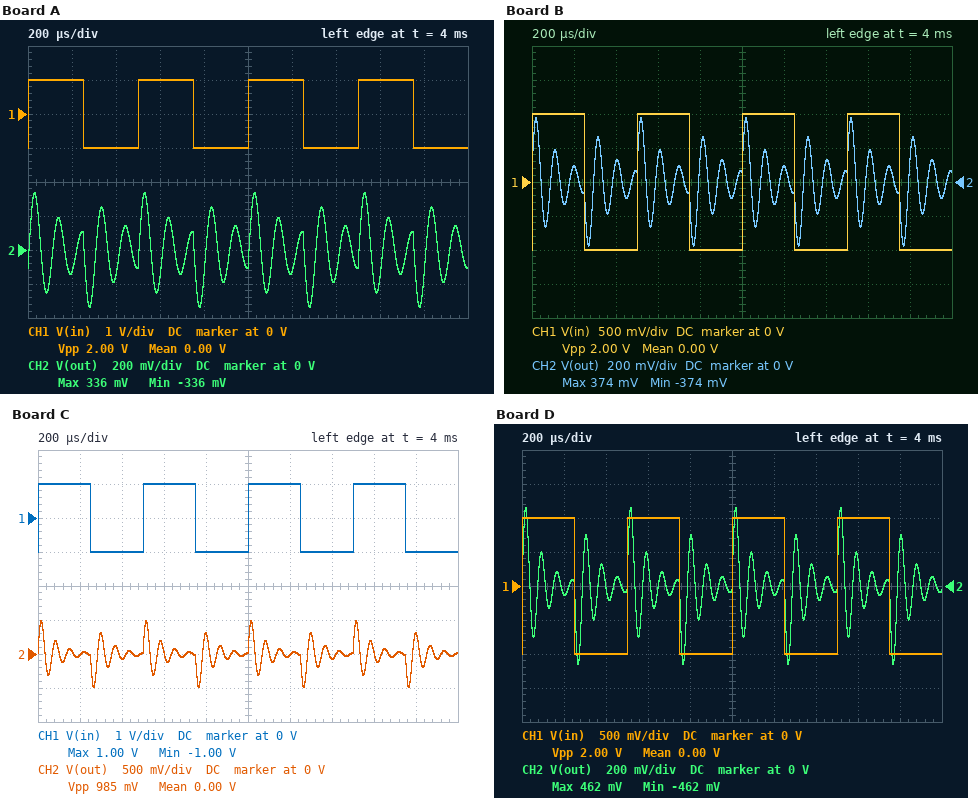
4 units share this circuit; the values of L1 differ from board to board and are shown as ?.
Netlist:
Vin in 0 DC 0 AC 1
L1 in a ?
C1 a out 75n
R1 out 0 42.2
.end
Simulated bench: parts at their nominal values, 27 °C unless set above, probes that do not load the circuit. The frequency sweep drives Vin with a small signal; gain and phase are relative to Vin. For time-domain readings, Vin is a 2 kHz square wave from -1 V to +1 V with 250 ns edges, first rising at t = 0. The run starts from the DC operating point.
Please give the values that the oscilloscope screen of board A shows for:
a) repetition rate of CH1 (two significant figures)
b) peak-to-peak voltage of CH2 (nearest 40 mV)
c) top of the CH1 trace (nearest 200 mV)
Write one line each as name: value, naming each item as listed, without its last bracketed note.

repetition rate of CH1: 2.0 kHz
peak-to-peak voltage of CH2: 680 mV
top of the CH1 trace: 1.0 V
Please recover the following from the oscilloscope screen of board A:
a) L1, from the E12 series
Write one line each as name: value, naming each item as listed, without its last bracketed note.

L1, from the E12 series: 3.9 mH
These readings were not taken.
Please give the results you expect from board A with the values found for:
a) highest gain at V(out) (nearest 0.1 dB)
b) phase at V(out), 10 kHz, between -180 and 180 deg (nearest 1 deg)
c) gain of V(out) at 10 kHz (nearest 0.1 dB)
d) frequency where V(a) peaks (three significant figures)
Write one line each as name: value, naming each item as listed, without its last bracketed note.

highest gain at V(out): 0 dB
phase at V(out), 10 kHz, between -180 and 180 deg: -38 deg
gain of V(out) at 10 kHz: -2.1 dB
frequency where V(a) peaks: 9.23 kHz
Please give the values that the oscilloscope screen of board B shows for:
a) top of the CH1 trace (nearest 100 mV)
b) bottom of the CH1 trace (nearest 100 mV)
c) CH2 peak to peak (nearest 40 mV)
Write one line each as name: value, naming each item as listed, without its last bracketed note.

top of the CH1 trace: 1.0 V
bottom of the CH1 trace: -1.0 V
CH2 peak to peak: 760 mV
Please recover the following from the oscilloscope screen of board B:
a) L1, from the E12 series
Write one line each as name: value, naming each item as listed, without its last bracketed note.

L1, from the E12 series: 2.7 mH
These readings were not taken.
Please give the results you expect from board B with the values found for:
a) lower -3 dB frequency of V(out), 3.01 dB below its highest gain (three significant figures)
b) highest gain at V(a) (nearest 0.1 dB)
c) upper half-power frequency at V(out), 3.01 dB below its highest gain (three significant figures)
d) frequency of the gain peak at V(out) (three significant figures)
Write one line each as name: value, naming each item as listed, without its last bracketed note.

lower -3 dB frequency of V(out), 3.01 dB below its highest gain: 10.0 kHz
highest gain at V(a): 13.3 dB
upper half-power frequency at V(out), 3.01 dB below its highest gain: 12.5 kHz
frequency of the gain peak at V(out): 11.2 kHz
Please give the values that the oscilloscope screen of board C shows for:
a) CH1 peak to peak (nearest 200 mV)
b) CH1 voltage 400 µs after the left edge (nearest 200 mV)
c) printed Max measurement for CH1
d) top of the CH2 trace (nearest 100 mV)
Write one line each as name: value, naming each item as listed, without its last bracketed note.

CH1 peak to peak: 2.0 V
CH1 voltage 400 µs after the left edge: -1.0 V
printed Max measurement for CH1: 1.00 V
top of the CH2 trace: 500 mV
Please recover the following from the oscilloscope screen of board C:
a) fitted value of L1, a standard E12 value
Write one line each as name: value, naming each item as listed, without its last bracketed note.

fitted value of L1, a standard E12 value: 1.5 mH
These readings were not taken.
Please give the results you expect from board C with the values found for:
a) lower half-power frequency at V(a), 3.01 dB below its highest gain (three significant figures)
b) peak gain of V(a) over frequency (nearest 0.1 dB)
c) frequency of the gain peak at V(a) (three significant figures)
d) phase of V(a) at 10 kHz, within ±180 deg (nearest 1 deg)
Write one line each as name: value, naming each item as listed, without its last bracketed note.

lower half-power frequency at V(a), 3.01 dB below its highest gain: 12.3 kHz
peak gain of V(a) over frequency: 11.0 dB
frequency of the gain peak at V(a): 14.7 kHz
phase of V(a) at 10 kHz, within ±180 deg: -8 deg
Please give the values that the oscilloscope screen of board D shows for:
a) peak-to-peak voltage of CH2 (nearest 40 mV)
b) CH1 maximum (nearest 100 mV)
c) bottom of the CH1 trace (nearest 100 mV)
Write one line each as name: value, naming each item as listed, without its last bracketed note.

peak-to-peak voltage of CH2: 920 mV
CH1 maximum: 1.0 V
bottom of the CH1 trace: -1.0 V
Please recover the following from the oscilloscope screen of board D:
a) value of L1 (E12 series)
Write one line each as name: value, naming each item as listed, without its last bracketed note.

value of L1: 1.8 mH
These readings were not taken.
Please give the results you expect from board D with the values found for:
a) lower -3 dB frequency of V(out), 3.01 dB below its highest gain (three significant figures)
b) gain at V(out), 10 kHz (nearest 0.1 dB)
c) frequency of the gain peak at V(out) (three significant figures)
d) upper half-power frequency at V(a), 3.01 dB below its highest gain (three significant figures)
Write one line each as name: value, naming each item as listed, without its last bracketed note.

lower -3 dB frequency of V(out), 3.01 dB below its highest gain: 12.0 kHz
gain at V(out), 10 kHz: -8.1 dB
frequency of the gain peak at V(out): 13.7 kHz
upper half-power frequency at V(a), 3.01 dB below its highest gain: 15.2 kHz
